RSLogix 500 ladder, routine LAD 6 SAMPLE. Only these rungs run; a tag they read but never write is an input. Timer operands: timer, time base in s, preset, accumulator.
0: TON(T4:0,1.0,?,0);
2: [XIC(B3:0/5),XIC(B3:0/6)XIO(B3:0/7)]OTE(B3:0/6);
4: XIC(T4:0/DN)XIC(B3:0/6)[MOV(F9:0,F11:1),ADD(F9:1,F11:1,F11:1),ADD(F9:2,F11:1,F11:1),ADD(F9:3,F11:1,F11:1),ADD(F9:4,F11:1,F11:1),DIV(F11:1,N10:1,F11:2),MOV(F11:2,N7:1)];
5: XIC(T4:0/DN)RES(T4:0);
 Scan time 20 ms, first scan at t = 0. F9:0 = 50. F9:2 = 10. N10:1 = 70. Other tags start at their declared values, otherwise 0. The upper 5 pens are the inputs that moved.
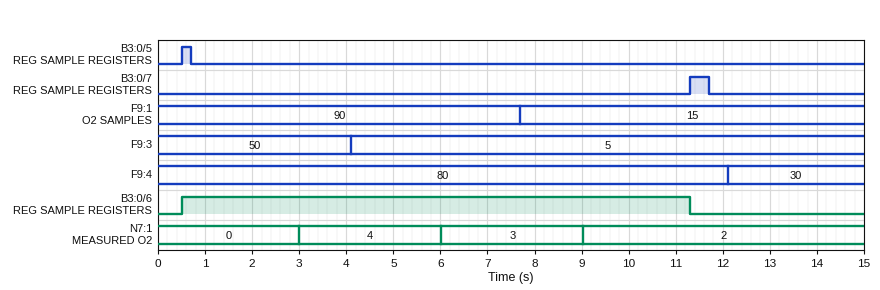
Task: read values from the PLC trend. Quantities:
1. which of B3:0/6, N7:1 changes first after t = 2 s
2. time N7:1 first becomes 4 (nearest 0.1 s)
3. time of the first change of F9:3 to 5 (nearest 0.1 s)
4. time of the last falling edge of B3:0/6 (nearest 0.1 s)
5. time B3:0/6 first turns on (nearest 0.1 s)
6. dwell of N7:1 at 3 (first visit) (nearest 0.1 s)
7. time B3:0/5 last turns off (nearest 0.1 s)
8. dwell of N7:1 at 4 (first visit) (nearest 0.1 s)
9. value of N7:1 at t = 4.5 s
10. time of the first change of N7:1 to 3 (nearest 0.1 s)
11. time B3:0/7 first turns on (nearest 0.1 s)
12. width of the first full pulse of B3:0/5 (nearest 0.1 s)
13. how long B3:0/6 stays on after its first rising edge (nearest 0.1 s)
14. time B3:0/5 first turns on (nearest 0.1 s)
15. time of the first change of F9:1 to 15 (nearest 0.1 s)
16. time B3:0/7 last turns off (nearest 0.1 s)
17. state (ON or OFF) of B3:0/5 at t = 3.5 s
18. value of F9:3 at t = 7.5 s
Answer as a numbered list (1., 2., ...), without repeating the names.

1. N7:1
2. 3.0 s
3. 4.1 s
4. 11.3 s
5. 0.5 s
6. 3.0 s
7. 0.7 s
8. 3.0 s
9. 4
10. 6.0 s
11. 11.3 s
12. 0.2 s
13. 10.8 s
14. 0.5 s
15. 7.7 s
16. 11.7 s
17. OFF
18. 5
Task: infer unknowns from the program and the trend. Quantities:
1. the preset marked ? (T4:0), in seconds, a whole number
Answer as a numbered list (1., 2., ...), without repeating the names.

1. 3 s
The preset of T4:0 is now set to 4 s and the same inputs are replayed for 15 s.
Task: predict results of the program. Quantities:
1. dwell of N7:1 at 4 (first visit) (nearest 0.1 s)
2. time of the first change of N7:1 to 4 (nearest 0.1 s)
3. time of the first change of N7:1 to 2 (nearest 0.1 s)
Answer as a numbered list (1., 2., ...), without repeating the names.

1. 4.0 s
2. 4.0 s
3. 8.0 s
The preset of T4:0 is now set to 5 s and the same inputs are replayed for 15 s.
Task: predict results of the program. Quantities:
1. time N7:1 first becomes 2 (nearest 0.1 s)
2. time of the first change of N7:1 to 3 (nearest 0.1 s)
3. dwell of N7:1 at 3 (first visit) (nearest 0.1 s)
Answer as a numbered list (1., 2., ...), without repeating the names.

1. 10.0 s
2. 5.0 s
3. 5.0 s
